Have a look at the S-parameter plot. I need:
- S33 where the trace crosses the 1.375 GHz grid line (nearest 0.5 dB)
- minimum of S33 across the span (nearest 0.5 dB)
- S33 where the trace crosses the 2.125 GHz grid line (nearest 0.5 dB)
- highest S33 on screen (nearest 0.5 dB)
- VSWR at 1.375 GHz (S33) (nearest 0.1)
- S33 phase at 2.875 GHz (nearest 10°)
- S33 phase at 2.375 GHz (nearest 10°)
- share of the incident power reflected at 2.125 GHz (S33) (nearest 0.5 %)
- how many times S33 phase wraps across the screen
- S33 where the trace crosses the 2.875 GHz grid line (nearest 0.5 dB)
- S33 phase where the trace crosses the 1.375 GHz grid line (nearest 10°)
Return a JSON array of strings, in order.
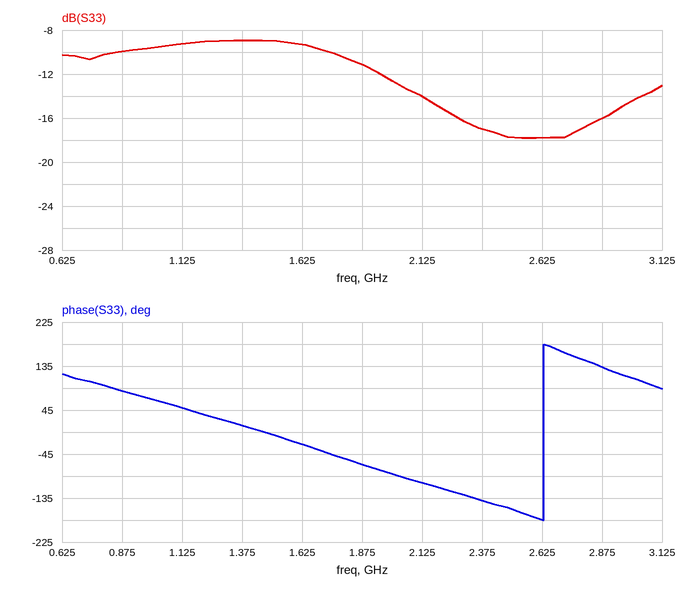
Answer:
["-9.0 dB", "-18.0 dB", "-14.0 dB", "-9.0 dB", "2.1", "130°", "-140°", "4.0 %", "1", "-16.0 dB", "10°"]
